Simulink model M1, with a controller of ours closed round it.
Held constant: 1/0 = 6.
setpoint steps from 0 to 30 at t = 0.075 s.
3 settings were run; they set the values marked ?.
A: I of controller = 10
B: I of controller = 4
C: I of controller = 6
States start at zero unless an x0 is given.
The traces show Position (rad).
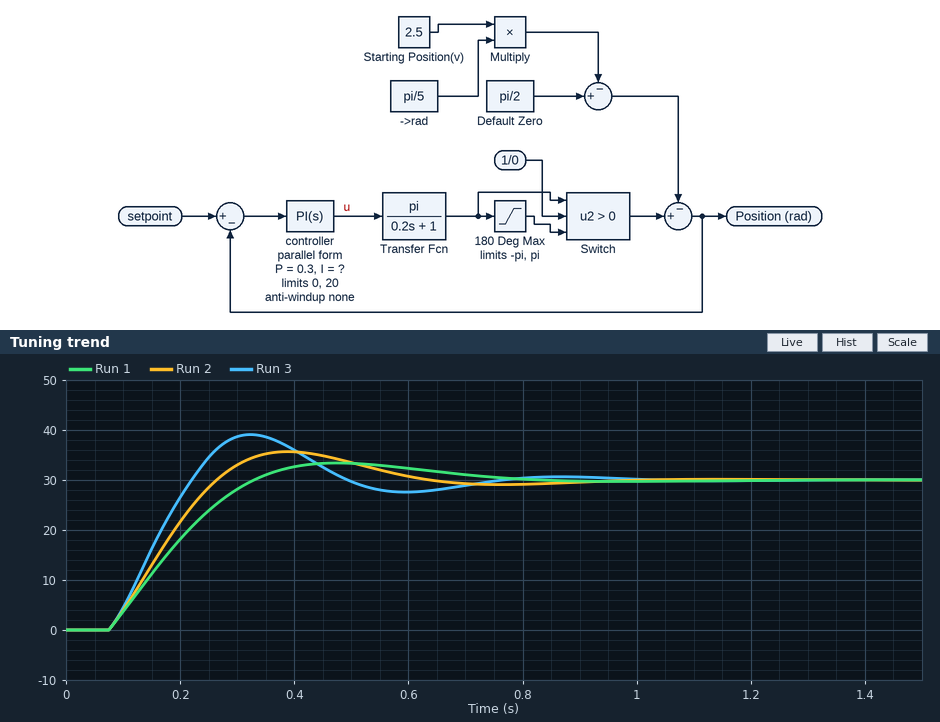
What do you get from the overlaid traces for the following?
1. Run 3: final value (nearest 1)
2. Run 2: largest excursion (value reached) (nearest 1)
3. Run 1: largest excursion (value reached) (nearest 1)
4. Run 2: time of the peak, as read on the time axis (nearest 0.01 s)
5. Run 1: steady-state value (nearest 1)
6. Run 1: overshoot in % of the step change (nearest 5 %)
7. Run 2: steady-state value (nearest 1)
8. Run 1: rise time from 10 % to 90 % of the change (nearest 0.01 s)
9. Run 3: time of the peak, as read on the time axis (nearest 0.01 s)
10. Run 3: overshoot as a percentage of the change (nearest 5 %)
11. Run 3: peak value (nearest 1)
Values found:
30
36
33
0.39 s
30
10 %
30
0.19 s
0.32 s
30 %
39
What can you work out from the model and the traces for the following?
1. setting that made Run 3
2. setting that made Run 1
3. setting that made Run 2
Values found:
A
B
C
